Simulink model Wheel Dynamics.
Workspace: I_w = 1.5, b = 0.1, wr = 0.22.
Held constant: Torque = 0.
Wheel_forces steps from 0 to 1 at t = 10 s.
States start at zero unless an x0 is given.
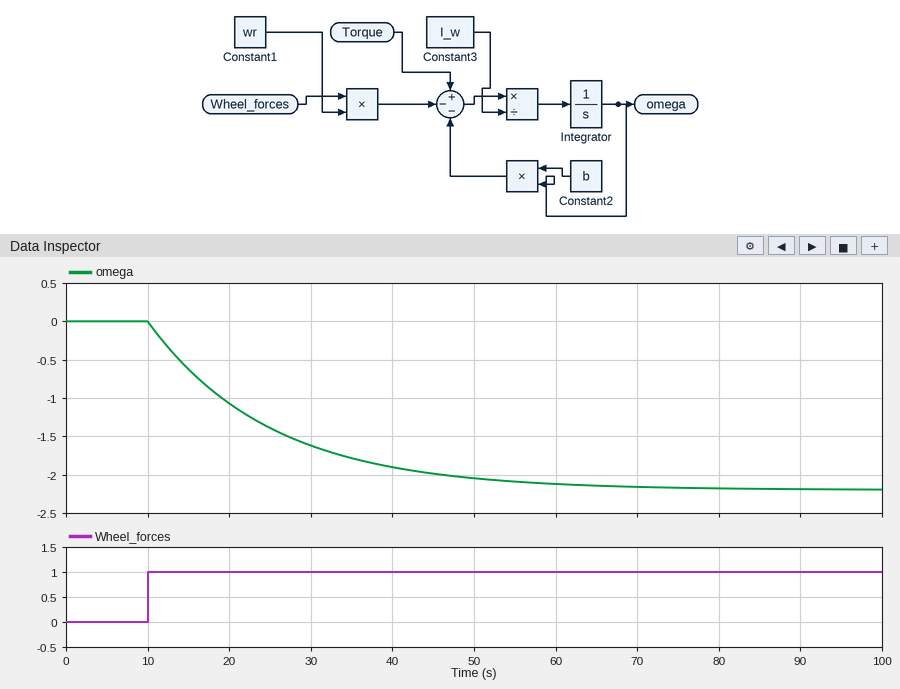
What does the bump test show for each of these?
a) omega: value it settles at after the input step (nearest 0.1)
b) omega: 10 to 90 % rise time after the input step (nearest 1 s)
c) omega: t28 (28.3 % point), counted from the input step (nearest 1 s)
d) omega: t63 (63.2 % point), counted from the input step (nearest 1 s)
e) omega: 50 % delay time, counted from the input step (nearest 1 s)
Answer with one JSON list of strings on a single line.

["-2.2", "33 s", "5 s", "15 s", "10 s"]
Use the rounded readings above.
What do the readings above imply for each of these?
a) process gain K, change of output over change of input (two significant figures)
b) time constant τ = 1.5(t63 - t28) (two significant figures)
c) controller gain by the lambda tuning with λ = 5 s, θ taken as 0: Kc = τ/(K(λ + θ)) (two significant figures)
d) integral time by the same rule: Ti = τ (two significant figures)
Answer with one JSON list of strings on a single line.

["-2.2", "15 s", "-1.4", "15 s"]
